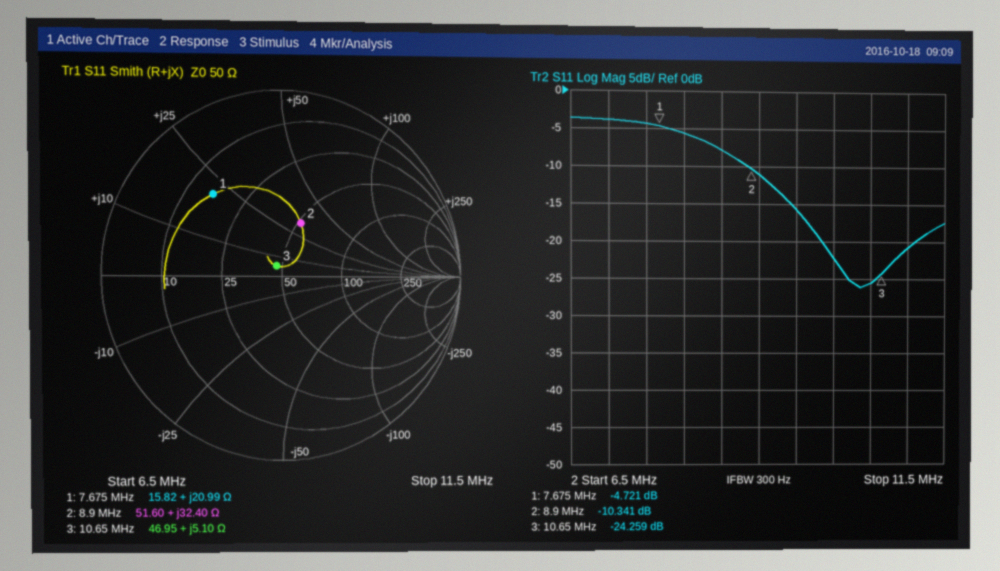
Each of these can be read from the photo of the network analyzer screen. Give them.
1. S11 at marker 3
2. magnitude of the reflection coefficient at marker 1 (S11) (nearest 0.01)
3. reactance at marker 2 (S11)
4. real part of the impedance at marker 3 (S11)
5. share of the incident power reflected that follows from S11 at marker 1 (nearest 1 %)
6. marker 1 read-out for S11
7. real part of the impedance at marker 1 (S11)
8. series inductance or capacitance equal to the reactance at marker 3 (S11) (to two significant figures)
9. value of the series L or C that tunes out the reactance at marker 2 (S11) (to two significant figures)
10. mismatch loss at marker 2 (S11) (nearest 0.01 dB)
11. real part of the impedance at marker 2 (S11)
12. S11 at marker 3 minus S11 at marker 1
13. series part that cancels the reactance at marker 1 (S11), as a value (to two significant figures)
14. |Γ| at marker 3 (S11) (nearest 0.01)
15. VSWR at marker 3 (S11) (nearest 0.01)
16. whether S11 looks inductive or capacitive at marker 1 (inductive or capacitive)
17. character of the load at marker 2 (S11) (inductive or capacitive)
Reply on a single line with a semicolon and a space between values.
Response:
-24.259 dB; 0.58; +32.40 Ω; 46.95 Ω; 34 %; -4.721 dB; 15.82 Ω; 76 nH; 550 pF; 0.42 dB; 51.60 Ω; -19.538 dB; 990 pF; 0.06; 1.13; inductive; inductive
